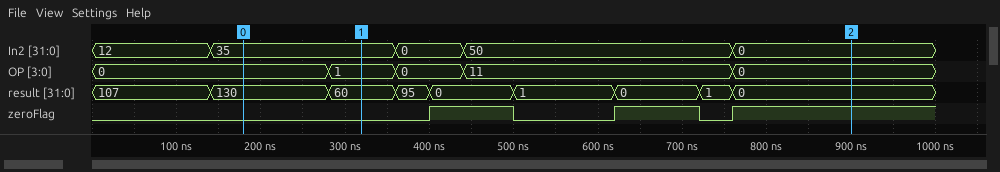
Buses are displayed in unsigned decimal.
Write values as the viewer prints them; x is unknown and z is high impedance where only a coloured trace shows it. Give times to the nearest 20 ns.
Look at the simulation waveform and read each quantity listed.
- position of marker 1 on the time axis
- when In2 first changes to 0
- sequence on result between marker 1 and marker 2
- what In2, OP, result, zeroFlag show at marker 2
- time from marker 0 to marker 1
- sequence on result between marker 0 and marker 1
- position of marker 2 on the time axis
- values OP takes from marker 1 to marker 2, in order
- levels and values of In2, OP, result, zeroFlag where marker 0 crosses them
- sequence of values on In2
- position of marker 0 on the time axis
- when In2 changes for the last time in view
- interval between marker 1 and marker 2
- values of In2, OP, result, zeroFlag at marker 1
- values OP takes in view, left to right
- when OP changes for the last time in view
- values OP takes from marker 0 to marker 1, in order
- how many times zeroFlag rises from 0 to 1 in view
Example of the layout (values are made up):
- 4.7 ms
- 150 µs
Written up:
- 320 ns
- 360 ns
- 60, 95, 0, 1, 0, 1, 0
- In2=0, OP=0, result=0, zeroFlag=1
- 140 ns
- 130, 60
- 900 ns
- 1, 0, 11, 0
- In2=35, OP=0, result=130, zeroFlag=0
- 12, 35, 0, 50, 0
- 180 ns
- 760 ns
- 580 ns
- In2=35, OP=1, result=60, zeroFlag=0
- 0, 1, 0, 11, 0
- 760 ns
- 0, 1
- 3
